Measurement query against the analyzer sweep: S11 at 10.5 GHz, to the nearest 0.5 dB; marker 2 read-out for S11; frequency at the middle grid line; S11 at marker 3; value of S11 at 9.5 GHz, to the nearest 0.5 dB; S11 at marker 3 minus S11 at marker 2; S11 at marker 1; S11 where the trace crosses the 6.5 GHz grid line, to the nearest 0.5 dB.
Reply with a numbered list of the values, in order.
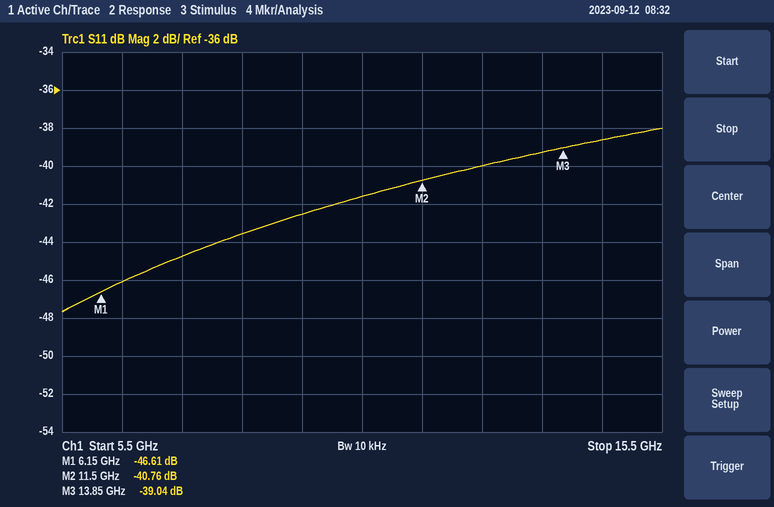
1. -41.5 dB
2. -40.76 dB
3. 10.5 GHz
4. -39.04 dB
5. -42.5 dB
6. 1.72 dB
7. -46.61 dB
8. -46.0 dB
